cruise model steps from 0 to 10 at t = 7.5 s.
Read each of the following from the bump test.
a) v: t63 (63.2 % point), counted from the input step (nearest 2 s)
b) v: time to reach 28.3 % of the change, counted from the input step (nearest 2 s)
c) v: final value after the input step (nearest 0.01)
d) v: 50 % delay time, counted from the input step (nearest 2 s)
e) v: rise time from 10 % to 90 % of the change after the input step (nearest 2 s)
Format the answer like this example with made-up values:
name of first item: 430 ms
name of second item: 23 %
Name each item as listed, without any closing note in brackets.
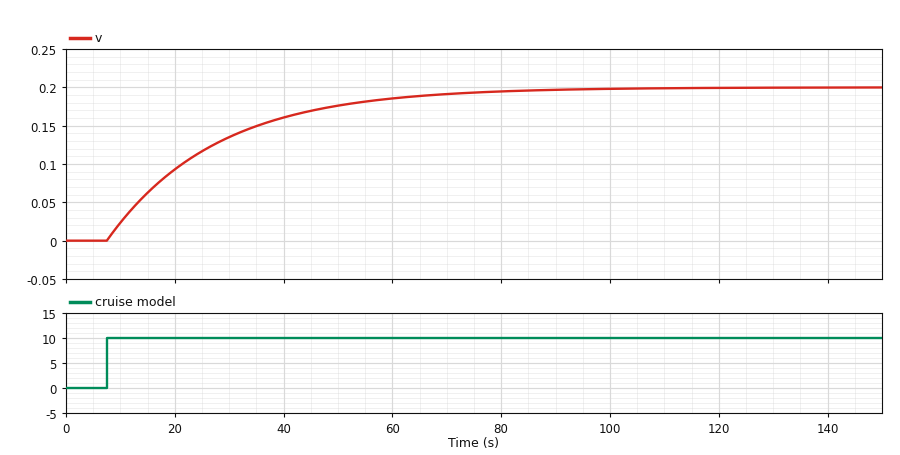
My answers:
v: t63 (63.2 % point), counted from the input step: 20 s
v: time to reach 28.3 % of the change, counted from the input step: 6 s
v: final value after the input step: 0.20
v: 50 % delay time, counted from the input step: 14 s
v: rise time from 10 % to 90 % of the change after the input step: 44 s
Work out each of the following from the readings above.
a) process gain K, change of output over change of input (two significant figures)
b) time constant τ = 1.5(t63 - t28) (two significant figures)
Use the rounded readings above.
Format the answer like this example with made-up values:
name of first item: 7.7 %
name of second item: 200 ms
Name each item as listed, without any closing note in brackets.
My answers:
process gain K, change of output over change of input: 0.020
time constant τ = 1.5(t63 - t28): 21 s
